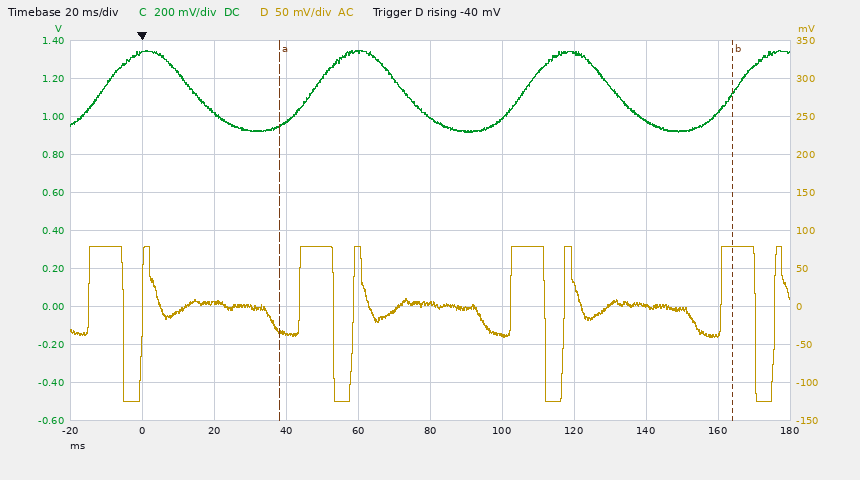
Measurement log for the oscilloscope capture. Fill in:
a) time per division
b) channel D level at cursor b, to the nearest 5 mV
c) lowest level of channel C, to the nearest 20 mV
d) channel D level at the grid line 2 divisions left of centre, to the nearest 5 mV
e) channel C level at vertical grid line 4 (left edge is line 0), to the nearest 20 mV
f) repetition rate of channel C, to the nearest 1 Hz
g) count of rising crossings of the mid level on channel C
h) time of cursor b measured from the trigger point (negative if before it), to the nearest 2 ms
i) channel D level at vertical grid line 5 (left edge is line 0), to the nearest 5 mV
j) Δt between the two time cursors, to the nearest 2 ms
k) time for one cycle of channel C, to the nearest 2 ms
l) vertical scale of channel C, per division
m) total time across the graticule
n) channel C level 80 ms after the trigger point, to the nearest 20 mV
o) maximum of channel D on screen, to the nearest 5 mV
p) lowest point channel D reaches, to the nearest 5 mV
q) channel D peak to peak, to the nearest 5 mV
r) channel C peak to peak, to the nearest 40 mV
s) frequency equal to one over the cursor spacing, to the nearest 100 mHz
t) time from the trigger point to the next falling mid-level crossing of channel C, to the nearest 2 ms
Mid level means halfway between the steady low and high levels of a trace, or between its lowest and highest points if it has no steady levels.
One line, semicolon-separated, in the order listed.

20 ms; 80 mV; 920 mV; -35 mV; 1.34 V; 17 Hz; 4; +164 ms; 5 mV; 126 ms; 58 ms; 200 mV; 200 ms; 1.00 V; 80 mV; -125 mV; 205 mV; 440 mV; 7.9 Hz; 14 ms
